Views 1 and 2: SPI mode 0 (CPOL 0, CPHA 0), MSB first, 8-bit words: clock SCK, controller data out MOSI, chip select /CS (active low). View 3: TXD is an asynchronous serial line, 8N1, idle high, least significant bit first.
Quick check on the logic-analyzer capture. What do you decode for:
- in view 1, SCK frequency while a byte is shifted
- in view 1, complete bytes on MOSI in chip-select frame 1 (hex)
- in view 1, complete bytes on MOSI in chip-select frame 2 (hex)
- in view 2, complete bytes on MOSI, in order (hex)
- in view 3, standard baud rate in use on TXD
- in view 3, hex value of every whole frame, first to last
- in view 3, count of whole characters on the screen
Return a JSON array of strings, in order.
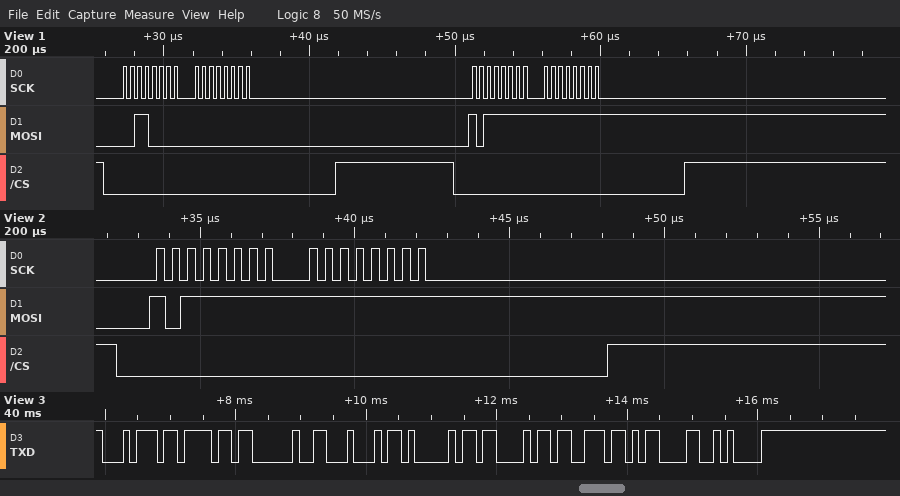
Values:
["2 MHz", "30 00", "BF FF", "BF FF", "9600 baud", "0x74 0x6F 0x20 0x44 0x41 0x43 0x73 0x0D 0x0A", "9"]
